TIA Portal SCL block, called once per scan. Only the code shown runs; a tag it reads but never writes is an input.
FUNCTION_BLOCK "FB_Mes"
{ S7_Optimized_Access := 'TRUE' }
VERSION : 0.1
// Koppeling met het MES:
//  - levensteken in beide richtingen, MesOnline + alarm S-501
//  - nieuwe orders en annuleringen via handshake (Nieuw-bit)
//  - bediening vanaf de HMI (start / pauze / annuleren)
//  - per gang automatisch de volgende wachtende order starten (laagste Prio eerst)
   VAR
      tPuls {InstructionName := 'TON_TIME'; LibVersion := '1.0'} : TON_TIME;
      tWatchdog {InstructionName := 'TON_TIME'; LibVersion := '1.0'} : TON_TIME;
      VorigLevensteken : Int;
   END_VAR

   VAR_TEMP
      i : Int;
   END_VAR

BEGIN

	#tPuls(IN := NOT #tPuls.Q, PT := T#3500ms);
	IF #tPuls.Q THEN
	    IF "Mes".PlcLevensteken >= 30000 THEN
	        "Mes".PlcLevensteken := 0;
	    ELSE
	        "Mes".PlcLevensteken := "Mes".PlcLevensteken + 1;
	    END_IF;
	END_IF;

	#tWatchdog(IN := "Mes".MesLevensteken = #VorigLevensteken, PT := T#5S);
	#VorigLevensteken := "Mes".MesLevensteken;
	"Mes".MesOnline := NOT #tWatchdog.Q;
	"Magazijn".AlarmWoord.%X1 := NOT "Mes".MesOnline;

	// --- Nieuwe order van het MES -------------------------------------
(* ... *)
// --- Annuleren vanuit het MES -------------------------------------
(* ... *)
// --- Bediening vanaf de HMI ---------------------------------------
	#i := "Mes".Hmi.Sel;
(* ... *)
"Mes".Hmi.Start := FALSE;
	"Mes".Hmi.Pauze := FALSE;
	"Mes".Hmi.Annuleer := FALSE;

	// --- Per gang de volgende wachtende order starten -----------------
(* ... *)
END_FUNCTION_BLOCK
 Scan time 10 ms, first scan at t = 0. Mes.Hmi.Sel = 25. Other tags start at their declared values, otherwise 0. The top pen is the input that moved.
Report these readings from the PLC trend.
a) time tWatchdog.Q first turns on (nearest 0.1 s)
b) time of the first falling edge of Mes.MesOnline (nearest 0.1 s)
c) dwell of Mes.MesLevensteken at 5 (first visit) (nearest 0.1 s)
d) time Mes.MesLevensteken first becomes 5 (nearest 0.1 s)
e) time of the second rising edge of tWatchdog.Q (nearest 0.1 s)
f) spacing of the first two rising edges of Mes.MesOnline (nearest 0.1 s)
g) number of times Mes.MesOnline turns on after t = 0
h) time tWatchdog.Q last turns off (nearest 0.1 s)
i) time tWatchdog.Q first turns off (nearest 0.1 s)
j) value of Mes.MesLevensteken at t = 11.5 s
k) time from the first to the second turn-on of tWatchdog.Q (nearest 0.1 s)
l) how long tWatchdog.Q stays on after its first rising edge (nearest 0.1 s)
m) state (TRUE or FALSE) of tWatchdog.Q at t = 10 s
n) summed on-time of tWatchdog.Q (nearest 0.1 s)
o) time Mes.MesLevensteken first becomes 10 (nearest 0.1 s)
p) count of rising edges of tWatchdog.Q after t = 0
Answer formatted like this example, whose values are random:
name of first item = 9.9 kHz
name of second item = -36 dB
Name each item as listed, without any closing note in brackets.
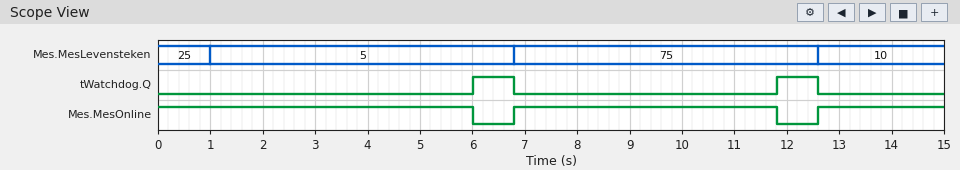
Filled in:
time tWatchdog.Q first turns on = 6.0 s
time of the first falling edge of Mes.MesOnline = 6.0 s
dwell of Mes.MesLevensteken at 5 (first visit) = 5.8 s
time Mes.MesLevensteken first becomes 5 = 1.0 s
time of the second rising edge of tWatchdog.Q = 11.8 s
spacing of the first two rising edges of Mes.MesOnline = 5.8 s
number of times Mes.MesOnline turns on after t = 0 = 2
time tWatchdog.Q last turns off = 12.6 s
time tWatchdog.Q first turns off = 6.8 s
value of Mes.MesLevensteken at t = 11.5 s = 75
time from the first to the second turn-on of tWatchdog.Q = 5.8 s
how long tWatchdog.Q stays on after its first rising edge = 0.8 s
state (TRUE or FALSE) of tWatchdog.Q at t = 10 s = FALSE
summed on-time of tWatchdog.Q = 1.6 s
time Mes.MesLevensteken first becomes 10 = 12.6 s
count of rising edges of tWatchdog.Q after t = 0 = 2
